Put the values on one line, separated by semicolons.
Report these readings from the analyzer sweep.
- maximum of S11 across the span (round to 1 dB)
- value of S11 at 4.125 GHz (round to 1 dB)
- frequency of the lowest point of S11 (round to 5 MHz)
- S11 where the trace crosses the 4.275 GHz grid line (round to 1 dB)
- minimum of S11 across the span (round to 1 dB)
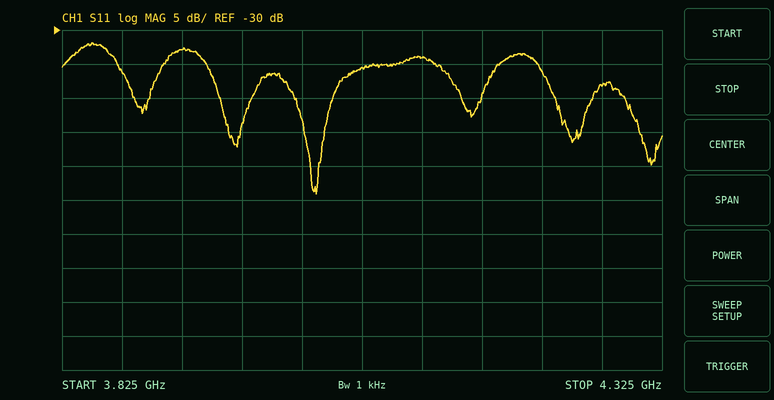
-32 dB; -34 dB; 4.035 GHz; -38 dB; -54 dB
